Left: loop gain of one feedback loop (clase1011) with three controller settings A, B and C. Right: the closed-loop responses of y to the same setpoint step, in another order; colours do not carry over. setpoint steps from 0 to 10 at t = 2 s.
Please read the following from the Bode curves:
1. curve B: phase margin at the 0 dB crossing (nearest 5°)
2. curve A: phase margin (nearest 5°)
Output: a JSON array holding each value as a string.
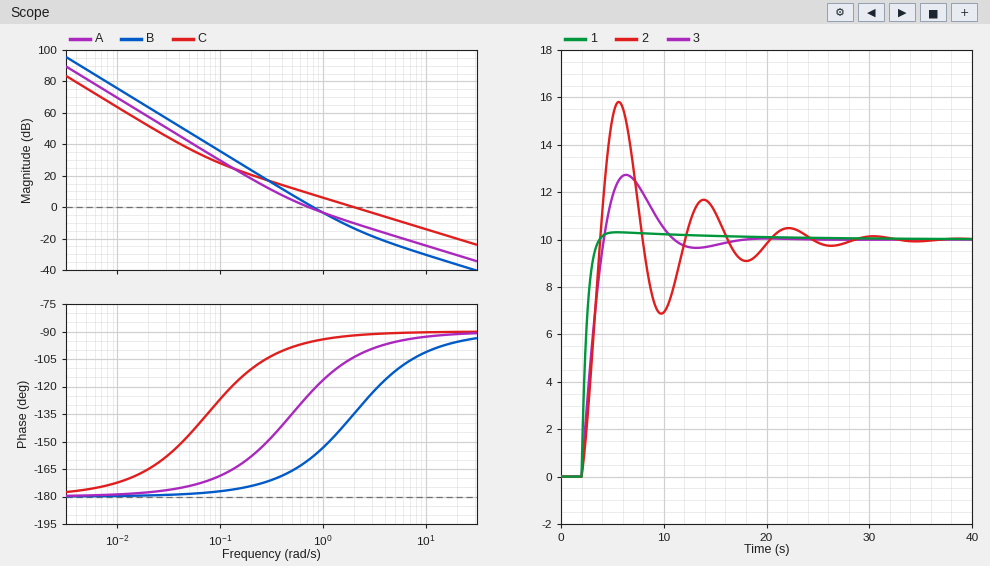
["20°", "55°"]
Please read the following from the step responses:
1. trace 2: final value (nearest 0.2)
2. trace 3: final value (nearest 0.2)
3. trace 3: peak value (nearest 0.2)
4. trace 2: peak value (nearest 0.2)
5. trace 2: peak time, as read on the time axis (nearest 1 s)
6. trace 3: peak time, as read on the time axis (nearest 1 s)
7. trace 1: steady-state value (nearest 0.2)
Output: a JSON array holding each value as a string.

["10.0", "10.0", "12.8", "15.8", "6 s", "6 s", "10.0"]
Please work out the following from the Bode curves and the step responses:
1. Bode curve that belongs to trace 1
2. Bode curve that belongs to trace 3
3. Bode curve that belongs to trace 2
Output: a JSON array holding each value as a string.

["C", "A", "B"]
